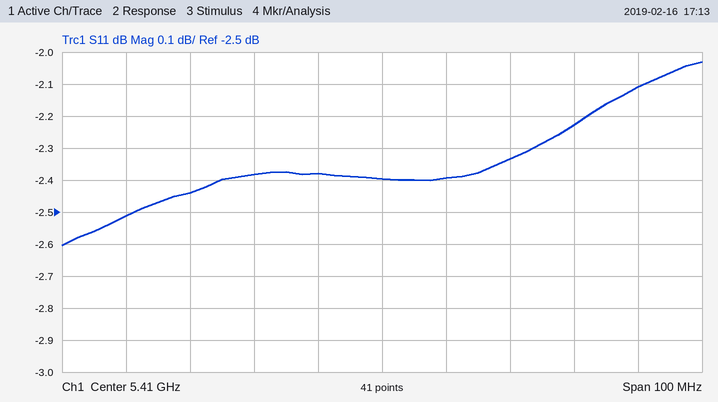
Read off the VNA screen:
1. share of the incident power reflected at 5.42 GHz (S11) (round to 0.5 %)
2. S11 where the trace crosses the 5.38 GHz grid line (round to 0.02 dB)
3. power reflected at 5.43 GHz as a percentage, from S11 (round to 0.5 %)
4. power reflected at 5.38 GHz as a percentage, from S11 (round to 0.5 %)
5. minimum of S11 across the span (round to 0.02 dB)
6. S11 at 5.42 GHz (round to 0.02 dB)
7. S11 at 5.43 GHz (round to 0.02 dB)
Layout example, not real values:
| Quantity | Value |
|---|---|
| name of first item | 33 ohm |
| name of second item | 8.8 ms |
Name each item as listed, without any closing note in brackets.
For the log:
| Quantity | Value |
|---|---|
| share of the incident power reflected at 5.42 GHz (S11) | 57.5 % |
| S11 where the trace crosses the 5.38 GHz grid line | -2.44 dB |
| power reflected at 5.43 GHz as a percentage, from S11 | 58.5 % |
| power reflected at 5.38 GHz as a percentage, from S11 | 57.0 % |
| minimum of S11 across the span | -2.60 dB |
| S11 at 5.42 GHz | -2.40 dB |
| S11 at 5.43 GHz | -2.34 dB |
